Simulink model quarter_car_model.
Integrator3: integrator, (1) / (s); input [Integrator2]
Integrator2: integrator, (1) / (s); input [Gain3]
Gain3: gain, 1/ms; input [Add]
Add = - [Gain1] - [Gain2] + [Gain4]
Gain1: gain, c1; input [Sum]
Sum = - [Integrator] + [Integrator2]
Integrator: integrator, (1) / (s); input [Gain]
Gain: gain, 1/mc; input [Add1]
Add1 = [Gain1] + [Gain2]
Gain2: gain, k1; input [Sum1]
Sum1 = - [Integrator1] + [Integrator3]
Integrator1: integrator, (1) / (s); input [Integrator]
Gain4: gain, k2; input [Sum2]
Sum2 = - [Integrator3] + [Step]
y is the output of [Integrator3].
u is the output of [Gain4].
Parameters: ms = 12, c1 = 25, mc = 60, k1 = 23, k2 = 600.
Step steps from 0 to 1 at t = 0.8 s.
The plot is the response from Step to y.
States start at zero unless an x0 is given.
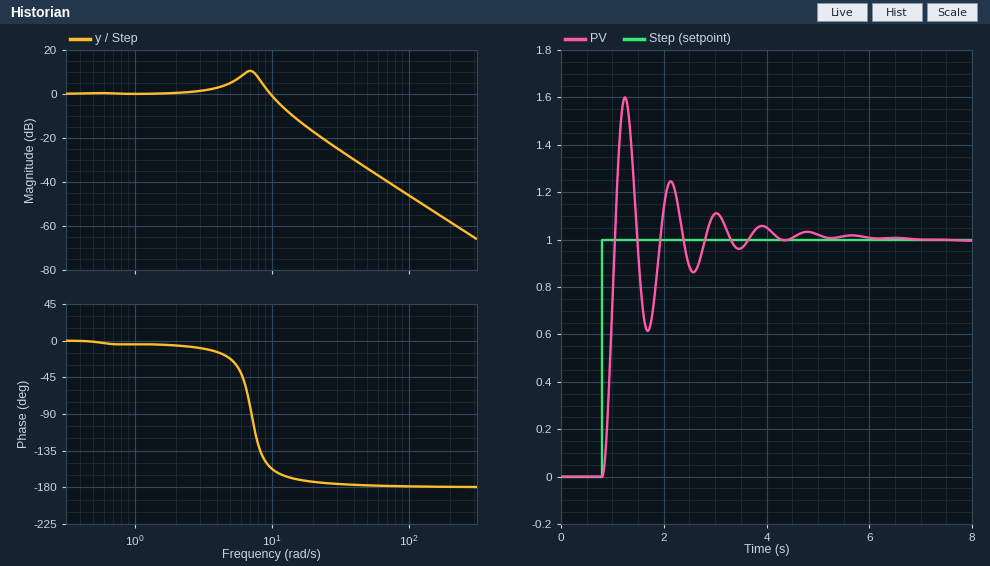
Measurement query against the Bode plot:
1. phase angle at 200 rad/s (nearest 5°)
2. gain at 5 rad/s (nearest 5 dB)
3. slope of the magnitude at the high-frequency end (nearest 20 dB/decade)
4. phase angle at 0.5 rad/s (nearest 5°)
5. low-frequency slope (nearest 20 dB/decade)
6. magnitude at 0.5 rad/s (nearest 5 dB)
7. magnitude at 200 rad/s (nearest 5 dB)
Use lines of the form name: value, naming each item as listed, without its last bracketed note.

phase angle at 200 rad/s: -180°
gain at 5 rad/s: 5 dB
slope of the magnitude at the high-frequency end: -40 dB/decade
phase angle at 0.5 rad/s: 0°
low-frequency slope: 0 dB/decade
magnitude at 0.5 rad/s: 0 dB
magnitude at 200 rad/s: -60 dB
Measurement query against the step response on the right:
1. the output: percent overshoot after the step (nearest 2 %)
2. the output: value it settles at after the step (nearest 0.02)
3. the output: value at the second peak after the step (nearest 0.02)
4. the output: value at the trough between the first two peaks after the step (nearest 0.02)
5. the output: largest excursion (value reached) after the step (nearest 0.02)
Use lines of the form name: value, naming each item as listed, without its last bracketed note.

the output: percent overshoot after the step: 60 %
the output: value it settles at after the step: 1.00
the output: value at the second peak after the step: 1.24
the output: value at the trough between the first two peaks after the step: 0.62
the output: largest excursion (value reached) after the step: 1.60
